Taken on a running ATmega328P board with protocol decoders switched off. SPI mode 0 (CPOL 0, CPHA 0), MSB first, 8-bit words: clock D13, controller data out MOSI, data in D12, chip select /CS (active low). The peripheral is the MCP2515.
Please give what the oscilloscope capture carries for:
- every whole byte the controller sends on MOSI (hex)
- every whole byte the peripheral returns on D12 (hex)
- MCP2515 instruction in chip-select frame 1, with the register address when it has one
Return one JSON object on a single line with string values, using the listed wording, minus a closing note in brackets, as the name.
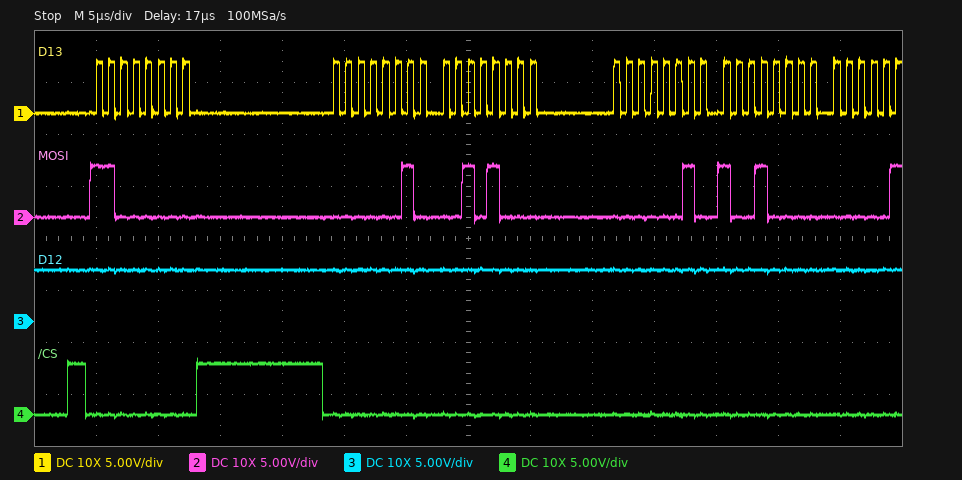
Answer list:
{"every whole byte the controller sends on MOSI": "0xC0 0x02 0x28 0x02 0x90", "every whole byte the peripheral returns on D12": "0xFF 0xFF 0xFF 0xFF 0xFF", "MCP2515 instruction in chip-select frame 1, with the register address when it has one": "RESET"}
